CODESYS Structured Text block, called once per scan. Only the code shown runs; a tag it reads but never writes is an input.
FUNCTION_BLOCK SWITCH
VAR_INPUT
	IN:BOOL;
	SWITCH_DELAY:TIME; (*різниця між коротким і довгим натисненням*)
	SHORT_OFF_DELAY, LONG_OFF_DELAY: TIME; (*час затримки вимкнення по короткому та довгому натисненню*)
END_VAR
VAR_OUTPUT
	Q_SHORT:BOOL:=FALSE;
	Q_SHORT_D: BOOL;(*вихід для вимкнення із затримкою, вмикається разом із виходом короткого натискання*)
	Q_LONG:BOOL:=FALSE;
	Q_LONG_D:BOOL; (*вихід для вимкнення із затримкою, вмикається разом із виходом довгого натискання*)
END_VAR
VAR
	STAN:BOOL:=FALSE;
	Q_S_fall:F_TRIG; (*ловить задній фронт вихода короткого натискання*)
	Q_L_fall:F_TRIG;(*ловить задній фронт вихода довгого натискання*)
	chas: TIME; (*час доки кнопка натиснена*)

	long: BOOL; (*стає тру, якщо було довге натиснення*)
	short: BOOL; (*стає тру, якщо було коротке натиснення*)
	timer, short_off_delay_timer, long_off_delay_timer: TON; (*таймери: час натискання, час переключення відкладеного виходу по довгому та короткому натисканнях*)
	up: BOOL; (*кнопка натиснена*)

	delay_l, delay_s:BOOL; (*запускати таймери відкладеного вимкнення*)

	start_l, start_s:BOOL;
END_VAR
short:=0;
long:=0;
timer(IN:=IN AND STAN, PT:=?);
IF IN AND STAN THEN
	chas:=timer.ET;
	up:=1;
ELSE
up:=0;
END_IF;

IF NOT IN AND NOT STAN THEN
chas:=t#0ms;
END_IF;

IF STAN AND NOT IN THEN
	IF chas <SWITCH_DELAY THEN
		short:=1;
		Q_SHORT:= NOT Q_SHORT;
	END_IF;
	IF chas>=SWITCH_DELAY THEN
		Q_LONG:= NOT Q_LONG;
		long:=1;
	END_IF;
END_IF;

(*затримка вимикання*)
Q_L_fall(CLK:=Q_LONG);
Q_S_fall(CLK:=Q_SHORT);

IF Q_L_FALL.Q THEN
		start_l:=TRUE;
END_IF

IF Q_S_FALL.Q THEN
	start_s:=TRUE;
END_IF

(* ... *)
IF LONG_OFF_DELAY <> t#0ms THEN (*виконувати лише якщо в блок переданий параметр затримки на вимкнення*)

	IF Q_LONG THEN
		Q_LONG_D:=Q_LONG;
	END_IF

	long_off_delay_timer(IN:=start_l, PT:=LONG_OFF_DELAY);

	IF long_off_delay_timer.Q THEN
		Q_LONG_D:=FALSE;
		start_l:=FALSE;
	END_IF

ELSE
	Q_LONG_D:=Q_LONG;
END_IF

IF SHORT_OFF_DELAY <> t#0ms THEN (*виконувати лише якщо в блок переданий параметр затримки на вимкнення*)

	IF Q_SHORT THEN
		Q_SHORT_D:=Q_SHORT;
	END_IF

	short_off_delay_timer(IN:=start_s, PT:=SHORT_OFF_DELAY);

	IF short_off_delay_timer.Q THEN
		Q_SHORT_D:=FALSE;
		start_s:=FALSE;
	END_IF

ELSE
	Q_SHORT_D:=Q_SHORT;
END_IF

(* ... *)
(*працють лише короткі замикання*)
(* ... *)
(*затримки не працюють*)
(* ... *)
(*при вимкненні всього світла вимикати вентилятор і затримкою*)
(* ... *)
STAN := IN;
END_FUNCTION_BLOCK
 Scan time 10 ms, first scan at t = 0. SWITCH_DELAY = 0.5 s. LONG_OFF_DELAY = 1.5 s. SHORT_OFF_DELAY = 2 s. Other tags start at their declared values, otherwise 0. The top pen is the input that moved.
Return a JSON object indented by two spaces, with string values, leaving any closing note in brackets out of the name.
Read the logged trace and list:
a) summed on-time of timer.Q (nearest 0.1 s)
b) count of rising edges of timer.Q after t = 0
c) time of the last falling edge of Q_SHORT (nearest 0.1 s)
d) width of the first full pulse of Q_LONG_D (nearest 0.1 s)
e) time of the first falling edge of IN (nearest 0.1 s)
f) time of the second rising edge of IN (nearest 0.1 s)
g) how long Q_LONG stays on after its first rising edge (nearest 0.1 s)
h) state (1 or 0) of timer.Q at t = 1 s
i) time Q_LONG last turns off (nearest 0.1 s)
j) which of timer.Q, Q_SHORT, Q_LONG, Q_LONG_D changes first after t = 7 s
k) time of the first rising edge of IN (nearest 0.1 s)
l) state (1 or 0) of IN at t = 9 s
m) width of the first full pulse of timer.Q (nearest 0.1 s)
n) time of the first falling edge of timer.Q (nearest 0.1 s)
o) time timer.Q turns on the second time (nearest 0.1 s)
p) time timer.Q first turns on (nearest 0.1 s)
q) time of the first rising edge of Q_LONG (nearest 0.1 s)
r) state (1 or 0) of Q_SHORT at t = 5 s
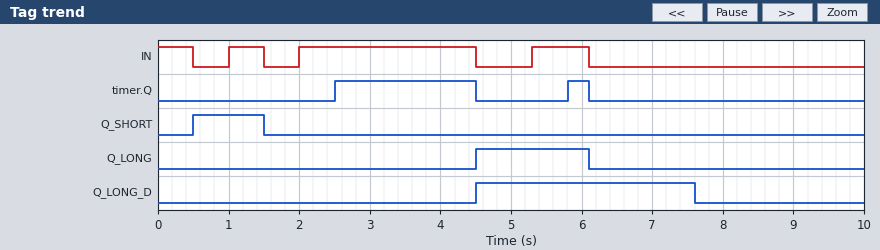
{
  "summed on-time of timer.Q": "2.3 s",
  "count of rising edges of timer.Q after t = 0": "2",
  "time of the last falling edge of Q_SHORT": "1.5 s",
  "width of the first full pulse of Q_LONG_D": "3.1 s",
  "time of the first falling edge of IN": "0.5 s",
  "time of the second rising edge of IN": "2.0 s",
  "how long Q_LONG stays on after its first rising edge": "1.6 s",
  "state (1 or 0) of timer.Q at t = 1 s": "0",
  "time Q_LONG last turns off": "6.1 s",
  "which of timer.Q, Q_SHORT, Q_LONG, Q_LONG_D changes first after t = 7 s": "Q_LONG_D",
  "time of the first rising edge of IN": "1.0 s",
  "state (1 or 0) of IN at t = 9 s": "0",
  "width of the first full pulse of timer.Q": "2.0 s",
  "time of the first falling edge of timer.Q": "4.5 s",
  "time timer.Q turns on the second time": "5.8 s",
  "time timer.Q first turns on": "2.5 s",
  "time of the first rising edge of Q_LONG": "4.5 s",
  "state (1 or 0) of Q_SHORT at t = 5 s": "0"
}
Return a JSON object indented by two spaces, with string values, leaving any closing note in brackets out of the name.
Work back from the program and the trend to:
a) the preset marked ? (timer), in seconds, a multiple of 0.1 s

{
  "the preset marked ? (timer), in seconds, a multiple of 0.1 s": "0.5 s"
}
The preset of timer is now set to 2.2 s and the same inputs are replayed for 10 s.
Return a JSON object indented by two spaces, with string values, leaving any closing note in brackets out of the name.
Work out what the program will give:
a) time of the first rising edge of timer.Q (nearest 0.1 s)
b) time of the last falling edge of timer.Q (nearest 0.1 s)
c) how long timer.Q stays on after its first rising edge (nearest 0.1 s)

{
  "time of the first rising edge of timer.Q": "4.2 s",
  "time of the last falling edge of timer.Q": "4.5 s",
  "how long timer.Q stays on after its first rising edge": "0.3 s"
}
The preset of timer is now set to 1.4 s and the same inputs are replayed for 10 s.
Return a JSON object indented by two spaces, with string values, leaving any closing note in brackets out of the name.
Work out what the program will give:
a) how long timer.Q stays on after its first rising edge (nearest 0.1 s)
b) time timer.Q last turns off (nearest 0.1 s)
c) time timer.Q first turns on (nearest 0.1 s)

{
  "how long timer.Q stays on after its first rising edge": "1.1 s",
  "time timer.Q last turns off": "4.5 s",
  "time timer.Q first turns on": "3.4 s"
}
